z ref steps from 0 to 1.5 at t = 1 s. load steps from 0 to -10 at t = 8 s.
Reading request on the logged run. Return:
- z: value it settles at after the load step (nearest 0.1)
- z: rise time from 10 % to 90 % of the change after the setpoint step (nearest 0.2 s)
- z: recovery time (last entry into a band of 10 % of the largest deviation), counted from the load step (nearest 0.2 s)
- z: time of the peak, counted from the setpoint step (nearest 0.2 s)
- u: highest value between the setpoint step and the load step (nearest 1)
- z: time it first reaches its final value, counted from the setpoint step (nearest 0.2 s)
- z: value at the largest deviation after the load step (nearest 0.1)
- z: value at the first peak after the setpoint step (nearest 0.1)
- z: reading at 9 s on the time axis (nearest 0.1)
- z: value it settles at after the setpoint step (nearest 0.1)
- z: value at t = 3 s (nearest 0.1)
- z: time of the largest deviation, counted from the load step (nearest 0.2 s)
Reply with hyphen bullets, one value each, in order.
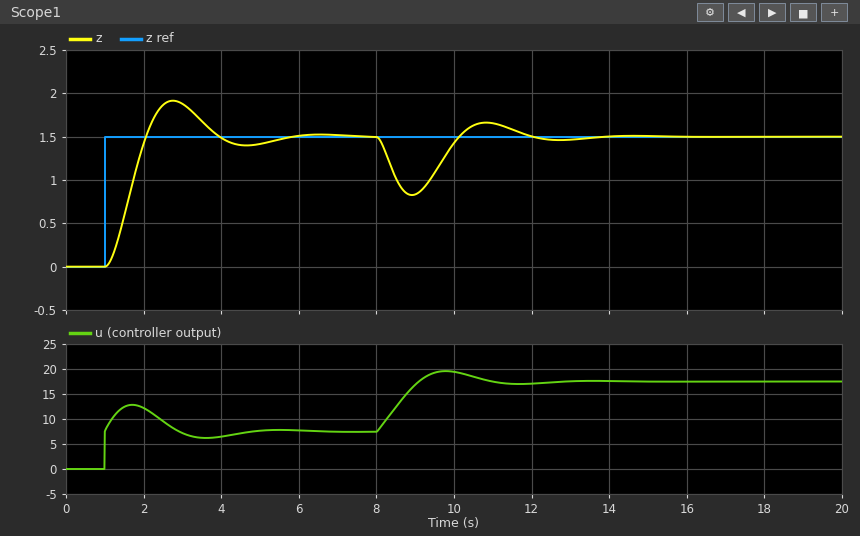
- 1.5
- 0.8 s
- 3.6 s
- 1.8 s
- 13
- 1.0 s
- 0.8
- 1.9
- 0.8
- 1.5
- 1.9
- 1.0 s
